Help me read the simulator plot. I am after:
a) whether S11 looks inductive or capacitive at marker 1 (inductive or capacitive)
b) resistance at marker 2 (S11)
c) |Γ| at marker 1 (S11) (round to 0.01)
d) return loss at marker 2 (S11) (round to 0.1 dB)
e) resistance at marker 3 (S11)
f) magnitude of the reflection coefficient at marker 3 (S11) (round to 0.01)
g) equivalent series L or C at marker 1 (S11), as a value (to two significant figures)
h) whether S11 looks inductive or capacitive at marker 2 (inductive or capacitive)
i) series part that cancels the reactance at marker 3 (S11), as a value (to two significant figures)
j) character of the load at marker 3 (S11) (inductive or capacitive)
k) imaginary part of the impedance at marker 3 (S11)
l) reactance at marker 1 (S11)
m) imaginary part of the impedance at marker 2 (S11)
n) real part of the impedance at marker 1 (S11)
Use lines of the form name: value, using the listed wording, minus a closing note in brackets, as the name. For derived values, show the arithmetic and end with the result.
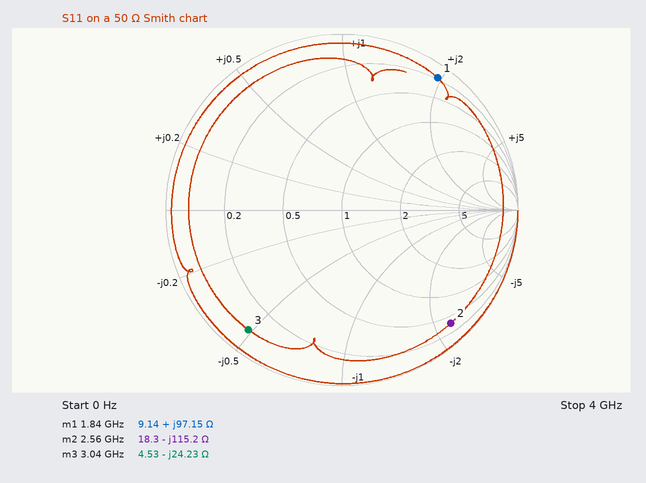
whether S11 looks inductive or capacitive at marker 1: inductive
resistance at marker 2: 18.3 Ω
|Γ| at marker 1 (S11): 0.93
return loss at marker 2 (S11): 1.0 dB
resistance at marker 3: 4.53 Ω
magnitude of the reflection coefficient at marker 3 (S11): 0.86
equivalent series L or C at marker 1 (S11), as a value: L = 97.15 Ω/(2π × 1.84 GHz) ≈ 8.4 nH
whether S11 looks inductive or capacitive at marker 2: capacitive
series part that cancels the reactance at marker 3 (S11), as a value: L = 24.23 Ω/(2π × 3.04 GHz) ≈ 1.3 nH
character of the load at marker 3 (S11): capacitive
imaginary part of the impedance at marker 3: -24.23 Ω
reactance at marker 1: +97.15 Ω
imaginary part of the impedance at marker 2: -115.2 Ω
real part of the impedance at marker 1: 9.14 Ω
